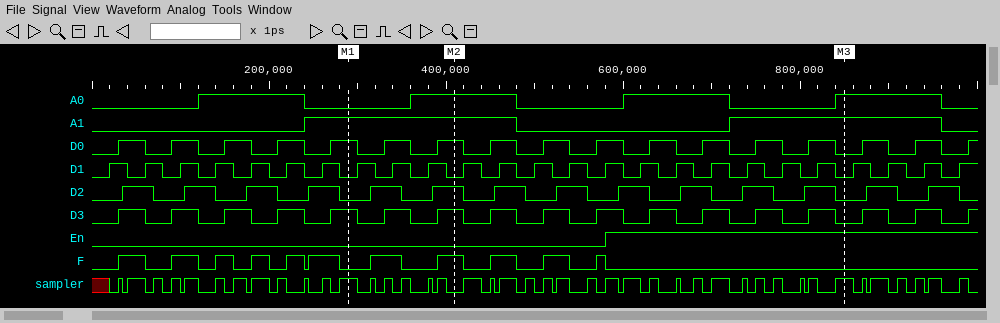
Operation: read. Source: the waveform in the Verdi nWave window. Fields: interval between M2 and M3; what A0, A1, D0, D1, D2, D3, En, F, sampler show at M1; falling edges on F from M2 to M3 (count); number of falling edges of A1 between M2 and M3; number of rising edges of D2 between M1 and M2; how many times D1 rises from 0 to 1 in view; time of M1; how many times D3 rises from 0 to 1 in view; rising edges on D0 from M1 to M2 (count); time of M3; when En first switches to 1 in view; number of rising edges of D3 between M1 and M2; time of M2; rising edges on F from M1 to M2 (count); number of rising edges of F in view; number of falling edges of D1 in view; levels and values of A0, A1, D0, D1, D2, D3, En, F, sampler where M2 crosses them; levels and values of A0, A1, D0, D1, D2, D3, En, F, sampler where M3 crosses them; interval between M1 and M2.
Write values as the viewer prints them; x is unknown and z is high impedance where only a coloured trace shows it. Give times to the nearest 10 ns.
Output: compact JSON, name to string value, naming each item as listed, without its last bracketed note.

{"interval between M2 and M3": "440 ns", "what A0, A1, D0, D1, D2, D3, En, F, sampler show at M1": "A0=0, A1=1, D0=1, D1=0, D2=0, D3=1, En=0, F=0, sampler=1", "falling edges on F from M2 to M3": "4", "number of falling edges of A1 between M2 and M3": "1", "number of rising edges of D2 between M1 and M2": "2", "how many times D1 rises from 0 to 1 in view": "25", "time of M1": "290 ns", "how many times D3 rises from 0 to 1 in view": "17", "rising edges on D0 from M1 to M2": "2", "time of M3": "850 ns", "when En first switches to 1 in view": "580 ns", "number of rising edges of D3 between M1 and M2": "2", "time of M2": "410 ns", "rising edges on F from M1 to M2": "2", "number of rising edges of F in view": "11", "number of falling edges of D1 in view": "24", "levels and values of A0, A1, D0, D1, D2, D3, En, F, sampler where M2 crosses them": "A0=1, A1=1, D0=1, D1=0, D2=1, D3=1, En=0, F=1, sampler=0", "levels and values of A0, A1, D0, D1, D2, D3, En, F, sampler where M3 crosses them": "A0=1, A1=1, D0=0, D1=0, D2=0, D3=0, En=1, F=0, sampler=1", "interval between M1 and M2": "120 ns"}
